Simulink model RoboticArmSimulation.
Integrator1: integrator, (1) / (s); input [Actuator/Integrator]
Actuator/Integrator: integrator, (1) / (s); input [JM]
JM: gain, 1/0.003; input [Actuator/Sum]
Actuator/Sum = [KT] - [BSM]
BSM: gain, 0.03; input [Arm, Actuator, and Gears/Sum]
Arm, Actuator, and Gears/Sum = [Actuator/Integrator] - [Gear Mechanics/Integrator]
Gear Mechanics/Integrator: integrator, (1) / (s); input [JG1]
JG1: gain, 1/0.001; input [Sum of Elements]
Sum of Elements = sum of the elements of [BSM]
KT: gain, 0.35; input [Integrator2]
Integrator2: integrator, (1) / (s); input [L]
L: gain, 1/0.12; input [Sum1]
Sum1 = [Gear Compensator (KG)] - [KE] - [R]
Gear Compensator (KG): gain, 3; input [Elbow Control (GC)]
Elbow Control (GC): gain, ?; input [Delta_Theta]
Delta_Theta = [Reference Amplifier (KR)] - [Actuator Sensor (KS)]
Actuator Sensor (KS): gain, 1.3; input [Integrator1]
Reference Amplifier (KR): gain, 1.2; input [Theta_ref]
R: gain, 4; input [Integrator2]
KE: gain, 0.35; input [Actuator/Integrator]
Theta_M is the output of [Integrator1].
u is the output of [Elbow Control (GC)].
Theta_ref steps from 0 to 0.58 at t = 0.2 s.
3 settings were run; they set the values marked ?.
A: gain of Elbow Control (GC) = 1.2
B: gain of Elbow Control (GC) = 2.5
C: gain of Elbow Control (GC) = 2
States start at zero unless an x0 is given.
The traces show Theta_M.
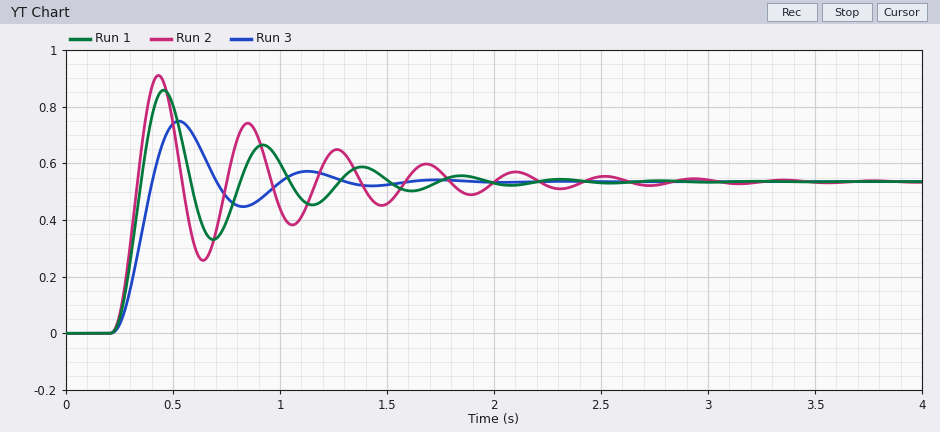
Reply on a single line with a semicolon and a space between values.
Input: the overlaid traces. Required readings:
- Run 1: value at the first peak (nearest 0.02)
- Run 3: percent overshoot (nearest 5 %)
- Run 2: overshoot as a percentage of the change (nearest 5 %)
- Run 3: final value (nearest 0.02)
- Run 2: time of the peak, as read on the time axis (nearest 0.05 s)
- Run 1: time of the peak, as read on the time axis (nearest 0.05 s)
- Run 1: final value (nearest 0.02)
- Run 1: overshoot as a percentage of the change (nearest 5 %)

0.86; 40 %; 70 %; 0.54; 0.45 s; 0.45 s; 0.54; 60 %
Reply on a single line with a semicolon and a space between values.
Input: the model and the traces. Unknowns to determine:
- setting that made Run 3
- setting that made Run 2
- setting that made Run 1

A; B; C
